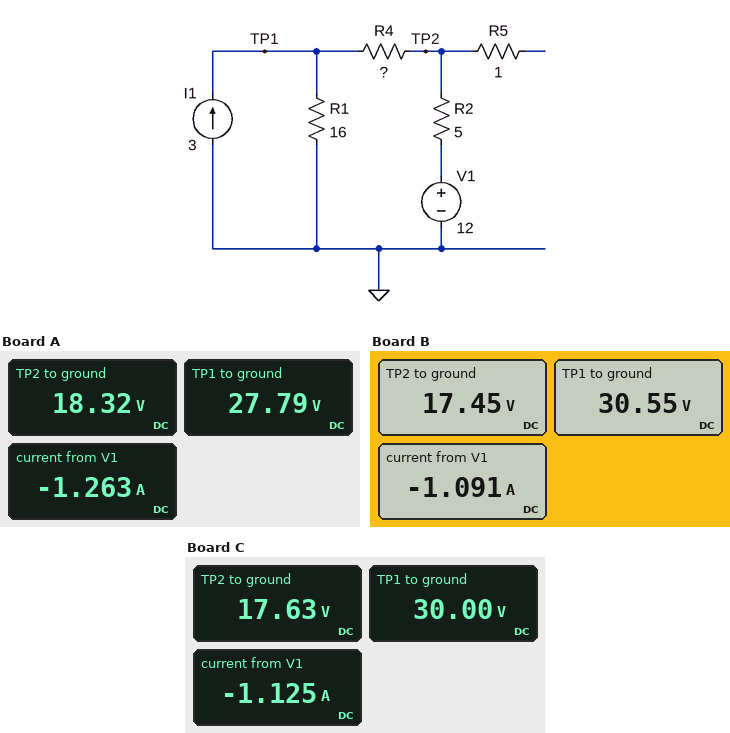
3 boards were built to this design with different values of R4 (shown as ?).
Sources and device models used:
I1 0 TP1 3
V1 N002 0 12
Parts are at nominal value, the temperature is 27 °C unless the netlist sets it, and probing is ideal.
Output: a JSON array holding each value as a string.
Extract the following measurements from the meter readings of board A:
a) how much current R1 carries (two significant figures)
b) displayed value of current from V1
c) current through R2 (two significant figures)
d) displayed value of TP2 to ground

["1.7 A", "-1.263 A", "1.3 A", "18.32 V"]
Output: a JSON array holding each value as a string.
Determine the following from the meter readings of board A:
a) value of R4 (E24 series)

["7.5 Ω"]
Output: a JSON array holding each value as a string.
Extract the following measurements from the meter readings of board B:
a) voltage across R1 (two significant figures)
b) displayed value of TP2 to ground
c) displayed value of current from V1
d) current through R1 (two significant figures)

["31 V", "17.45 V", "-1.091 A", "1.9 A"]
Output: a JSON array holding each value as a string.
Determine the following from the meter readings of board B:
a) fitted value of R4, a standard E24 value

["12 Ω"]
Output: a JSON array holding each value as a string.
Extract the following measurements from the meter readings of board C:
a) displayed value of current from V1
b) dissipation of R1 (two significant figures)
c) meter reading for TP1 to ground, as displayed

["-1.125 A", "56 W", "30.00 V"]
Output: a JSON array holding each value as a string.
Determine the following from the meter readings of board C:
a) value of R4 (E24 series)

["11 Ω"]
